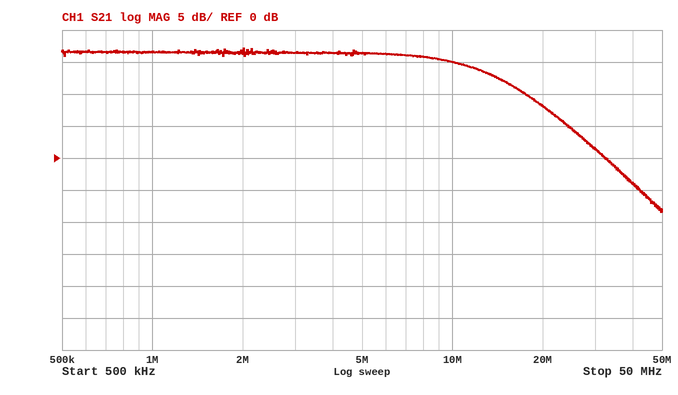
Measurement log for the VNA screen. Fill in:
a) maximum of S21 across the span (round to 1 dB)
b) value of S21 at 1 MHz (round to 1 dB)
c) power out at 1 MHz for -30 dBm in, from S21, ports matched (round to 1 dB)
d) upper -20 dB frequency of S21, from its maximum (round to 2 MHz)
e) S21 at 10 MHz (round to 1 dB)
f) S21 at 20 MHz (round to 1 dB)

17 dB
17 dB
-13 dBm
38 MHz
15 dB
8 dB
